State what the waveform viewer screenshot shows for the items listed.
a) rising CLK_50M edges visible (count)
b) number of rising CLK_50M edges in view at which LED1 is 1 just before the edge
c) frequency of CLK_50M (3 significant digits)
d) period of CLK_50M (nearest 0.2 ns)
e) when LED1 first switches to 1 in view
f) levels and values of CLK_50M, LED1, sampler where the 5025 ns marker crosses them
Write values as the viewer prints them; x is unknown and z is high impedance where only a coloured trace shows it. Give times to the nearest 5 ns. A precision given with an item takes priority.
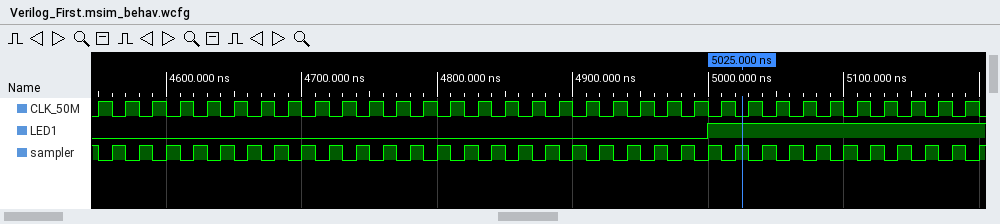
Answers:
33
10
50.0 MHz
20 ns
5000 ns
CLK_50M=0, LED1=1, sampler=1
